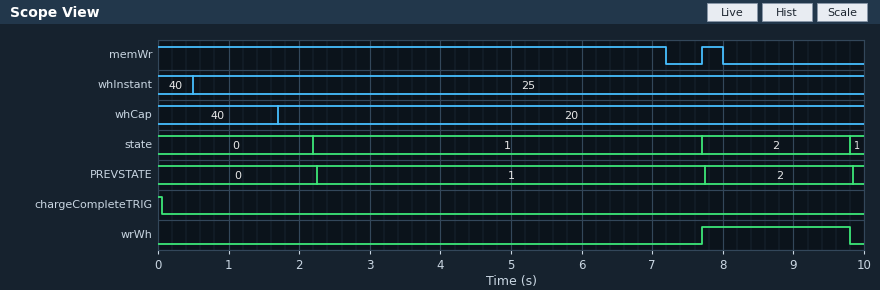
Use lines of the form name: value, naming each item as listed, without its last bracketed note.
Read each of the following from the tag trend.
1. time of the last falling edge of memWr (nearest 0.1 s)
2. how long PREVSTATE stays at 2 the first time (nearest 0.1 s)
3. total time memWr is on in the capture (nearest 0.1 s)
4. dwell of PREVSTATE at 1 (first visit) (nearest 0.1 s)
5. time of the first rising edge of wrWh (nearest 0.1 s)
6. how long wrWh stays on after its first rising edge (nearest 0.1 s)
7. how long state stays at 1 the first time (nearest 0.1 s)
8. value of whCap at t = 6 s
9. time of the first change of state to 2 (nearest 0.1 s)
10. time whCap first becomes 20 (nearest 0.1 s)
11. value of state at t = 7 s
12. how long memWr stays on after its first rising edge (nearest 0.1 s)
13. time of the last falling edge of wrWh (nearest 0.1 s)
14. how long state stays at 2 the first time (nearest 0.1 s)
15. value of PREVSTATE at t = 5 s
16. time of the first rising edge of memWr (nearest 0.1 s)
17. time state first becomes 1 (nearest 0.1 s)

time of the last falling edge of memWr: 8.0 s
how long PREVSTATE stays at 2 the first time: 2.1 s
total time memWr is on in the capture: 7.5 s
dwell of PREVSTATE at 1 (first visit): 5.5 s
time of the first rising edge of wrWh: 7.7 s
how long wrWh stays on after its first rising edge: 2.1 s
how long state stays at 1 the first time: 5.5 s
value of whCap at t = 6 s: 20
time of the first change of state to 2: 7.7 s
time whCap first becomes 20: 1.7 s
value of state at t = 7 s: 1
how long memWr stays on after its first rising edge: 0.3 s
time of the last falling edge of wrWh: 9.8 s
how long state stays at 2 the first time: 2.1 s
value of PREVSTATE at t = 5 s: 1
time of the first rising edge of memWr: 7.7 s
time state first becomes 1: 2.2 s
